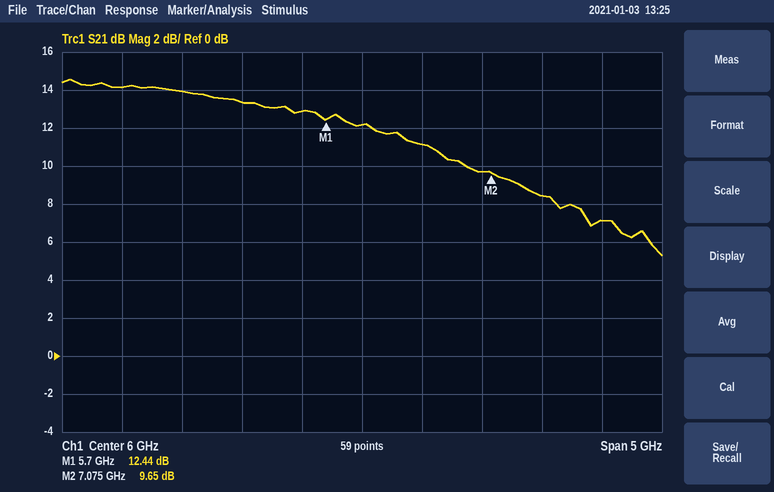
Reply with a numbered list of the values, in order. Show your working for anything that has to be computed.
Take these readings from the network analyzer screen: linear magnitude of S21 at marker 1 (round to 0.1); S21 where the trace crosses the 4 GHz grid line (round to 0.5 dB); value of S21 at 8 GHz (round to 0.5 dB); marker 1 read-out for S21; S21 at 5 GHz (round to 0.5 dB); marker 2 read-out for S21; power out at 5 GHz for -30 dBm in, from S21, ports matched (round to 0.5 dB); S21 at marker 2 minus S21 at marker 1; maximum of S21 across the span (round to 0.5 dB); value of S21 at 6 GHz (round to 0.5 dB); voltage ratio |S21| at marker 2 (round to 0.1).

1. 10^(12.44/20) ≈ 4.2
2. 14.0 dB
3. 7.0 dB
4. 12.44 dB
5. 13.5 dB
6. 9.65 dB
7. -30 dBm + (13.5 dB) = -16.5 dBm
8. 9.65 − (12.44) = -2.79 dB
9. 14.5 dB
10. 12.0 dB
11. 10^(9.65/20) ≈ 3.0
